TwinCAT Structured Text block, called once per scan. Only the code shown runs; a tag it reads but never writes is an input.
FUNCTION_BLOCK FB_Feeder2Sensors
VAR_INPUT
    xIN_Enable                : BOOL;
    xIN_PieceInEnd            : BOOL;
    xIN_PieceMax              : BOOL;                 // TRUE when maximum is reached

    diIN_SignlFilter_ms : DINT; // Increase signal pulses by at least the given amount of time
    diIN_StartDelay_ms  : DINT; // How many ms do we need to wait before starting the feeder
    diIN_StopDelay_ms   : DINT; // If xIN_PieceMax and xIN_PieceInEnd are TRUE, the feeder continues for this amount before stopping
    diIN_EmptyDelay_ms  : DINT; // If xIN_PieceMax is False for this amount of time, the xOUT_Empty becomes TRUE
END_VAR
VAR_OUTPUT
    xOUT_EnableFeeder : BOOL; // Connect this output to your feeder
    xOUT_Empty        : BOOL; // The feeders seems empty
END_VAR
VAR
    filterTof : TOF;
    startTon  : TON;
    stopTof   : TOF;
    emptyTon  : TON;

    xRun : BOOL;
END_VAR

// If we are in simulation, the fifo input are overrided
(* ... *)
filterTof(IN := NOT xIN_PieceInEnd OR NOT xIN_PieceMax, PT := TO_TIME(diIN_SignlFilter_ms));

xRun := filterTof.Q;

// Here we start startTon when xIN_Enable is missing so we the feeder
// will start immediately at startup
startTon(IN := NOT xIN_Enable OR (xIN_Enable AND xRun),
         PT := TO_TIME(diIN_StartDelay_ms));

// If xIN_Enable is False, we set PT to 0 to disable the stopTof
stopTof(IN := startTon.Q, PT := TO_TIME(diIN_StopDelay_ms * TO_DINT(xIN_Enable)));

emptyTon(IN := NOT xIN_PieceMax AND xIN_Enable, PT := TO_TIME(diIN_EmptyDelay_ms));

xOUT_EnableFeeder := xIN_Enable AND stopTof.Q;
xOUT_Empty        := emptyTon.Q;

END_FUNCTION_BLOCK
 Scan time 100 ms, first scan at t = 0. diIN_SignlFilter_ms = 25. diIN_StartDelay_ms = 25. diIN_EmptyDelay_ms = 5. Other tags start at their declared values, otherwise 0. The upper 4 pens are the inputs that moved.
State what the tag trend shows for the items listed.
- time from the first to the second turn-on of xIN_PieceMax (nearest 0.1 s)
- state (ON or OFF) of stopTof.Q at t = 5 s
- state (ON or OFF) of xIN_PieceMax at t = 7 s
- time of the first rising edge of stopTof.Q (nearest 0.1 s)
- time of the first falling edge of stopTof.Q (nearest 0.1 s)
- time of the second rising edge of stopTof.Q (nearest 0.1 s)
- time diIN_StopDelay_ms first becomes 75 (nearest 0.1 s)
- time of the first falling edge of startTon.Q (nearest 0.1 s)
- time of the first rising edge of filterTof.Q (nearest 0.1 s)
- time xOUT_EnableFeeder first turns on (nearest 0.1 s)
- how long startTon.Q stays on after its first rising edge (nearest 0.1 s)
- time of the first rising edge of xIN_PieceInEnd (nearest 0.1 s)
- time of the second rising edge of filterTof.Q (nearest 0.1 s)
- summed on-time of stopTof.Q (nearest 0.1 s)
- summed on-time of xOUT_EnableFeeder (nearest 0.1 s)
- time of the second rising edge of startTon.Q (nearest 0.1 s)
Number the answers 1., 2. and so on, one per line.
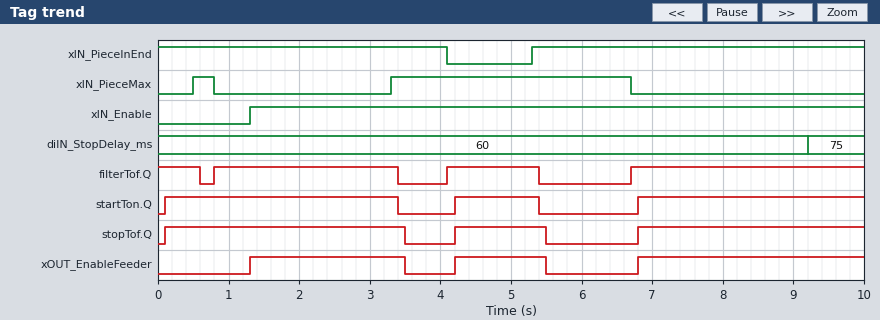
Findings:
1. 2.8 s
2. ON
3. OFF
4. 0.1 s
5. 3.5 s
6. 4.2 s
7. 9.2 s
8. 3.4 s
9. 0.8 s
10. 1.3 s
11. 3.3 s
12. 5.3 s
13. 4.1 s
14. 7.9 s
15. 6.7 s
16. 4.2 s
